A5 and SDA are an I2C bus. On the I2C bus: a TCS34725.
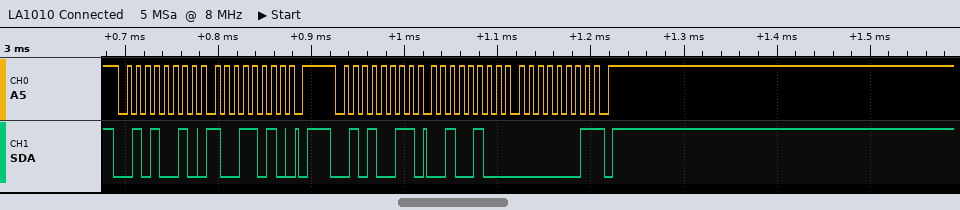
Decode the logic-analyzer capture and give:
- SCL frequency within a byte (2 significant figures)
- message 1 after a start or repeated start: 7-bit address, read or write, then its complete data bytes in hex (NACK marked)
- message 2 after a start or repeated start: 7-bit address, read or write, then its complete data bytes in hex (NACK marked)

100 kHz
0x29 write: 9A
0x29 read: 24 01 NACK
